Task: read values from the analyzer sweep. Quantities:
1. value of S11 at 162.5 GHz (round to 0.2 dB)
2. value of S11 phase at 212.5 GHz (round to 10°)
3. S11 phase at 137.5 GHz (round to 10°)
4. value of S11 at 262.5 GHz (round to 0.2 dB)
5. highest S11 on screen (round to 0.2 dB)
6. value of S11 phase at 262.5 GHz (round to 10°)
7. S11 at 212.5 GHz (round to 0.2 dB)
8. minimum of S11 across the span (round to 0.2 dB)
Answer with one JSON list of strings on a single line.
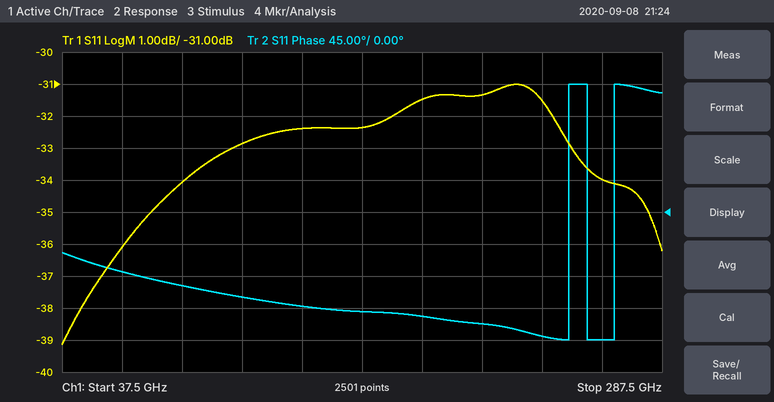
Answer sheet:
["-32.4 dB", "-160°", "-130°", "-34.0 dB", "-31.0 dB", "-180°", "-31.4 dB", "-39.2 dB"]
